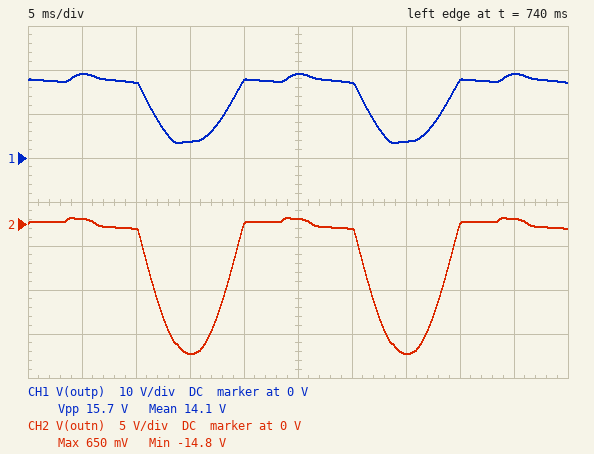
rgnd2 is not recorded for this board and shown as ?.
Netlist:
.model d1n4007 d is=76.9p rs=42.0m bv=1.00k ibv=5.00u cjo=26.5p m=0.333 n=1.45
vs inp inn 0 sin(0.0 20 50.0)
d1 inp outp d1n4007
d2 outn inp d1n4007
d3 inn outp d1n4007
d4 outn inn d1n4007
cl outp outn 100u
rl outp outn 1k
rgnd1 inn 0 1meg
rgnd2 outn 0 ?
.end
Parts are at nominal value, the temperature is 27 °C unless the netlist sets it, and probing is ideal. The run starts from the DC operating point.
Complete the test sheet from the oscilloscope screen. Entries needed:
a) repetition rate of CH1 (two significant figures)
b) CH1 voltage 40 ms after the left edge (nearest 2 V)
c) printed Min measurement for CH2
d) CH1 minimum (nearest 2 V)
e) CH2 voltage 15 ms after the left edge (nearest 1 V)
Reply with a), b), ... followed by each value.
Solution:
a) 50 Hz
b) 18 V
c) -14.8 V
d) 4 V
e) -15 V
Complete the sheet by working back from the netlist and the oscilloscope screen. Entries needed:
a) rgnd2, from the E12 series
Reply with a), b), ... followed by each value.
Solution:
a) 3.3 MΩ
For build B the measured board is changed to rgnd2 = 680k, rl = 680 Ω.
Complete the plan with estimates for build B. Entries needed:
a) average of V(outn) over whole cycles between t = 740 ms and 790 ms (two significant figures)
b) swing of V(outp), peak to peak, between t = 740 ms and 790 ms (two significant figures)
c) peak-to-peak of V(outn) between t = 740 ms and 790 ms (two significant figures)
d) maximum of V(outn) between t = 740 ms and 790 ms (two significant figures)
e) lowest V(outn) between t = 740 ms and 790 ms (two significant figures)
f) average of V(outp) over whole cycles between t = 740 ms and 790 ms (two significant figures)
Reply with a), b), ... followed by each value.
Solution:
a) -2.4 V
b) 9.3 V
c) 8.1 V
d) 340 mV
e) -7.8 V
f) 15 V
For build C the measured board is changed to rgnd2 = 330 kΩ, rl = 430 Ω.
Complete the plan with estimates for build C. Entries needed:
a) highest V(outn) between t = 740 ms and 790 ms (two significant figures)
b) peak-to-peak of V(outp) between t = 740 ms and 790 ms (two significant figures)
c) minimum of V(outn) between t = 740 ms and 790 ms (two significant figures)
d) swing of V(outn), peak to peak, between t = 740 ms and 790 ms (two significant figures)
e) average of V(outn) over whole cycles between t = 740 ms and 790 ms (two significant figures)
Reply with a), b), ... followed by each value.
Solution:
a) 210 mV
b) 7.3 V
c) -4.8 V
d) 5.0 V
e) -1.5 V
